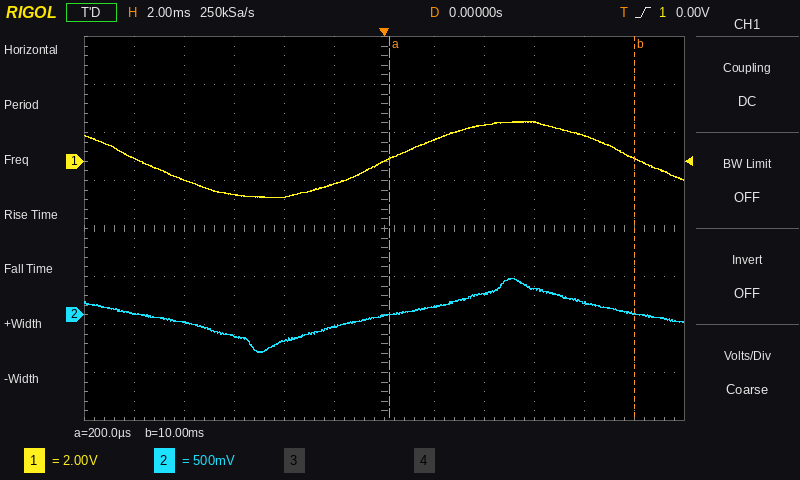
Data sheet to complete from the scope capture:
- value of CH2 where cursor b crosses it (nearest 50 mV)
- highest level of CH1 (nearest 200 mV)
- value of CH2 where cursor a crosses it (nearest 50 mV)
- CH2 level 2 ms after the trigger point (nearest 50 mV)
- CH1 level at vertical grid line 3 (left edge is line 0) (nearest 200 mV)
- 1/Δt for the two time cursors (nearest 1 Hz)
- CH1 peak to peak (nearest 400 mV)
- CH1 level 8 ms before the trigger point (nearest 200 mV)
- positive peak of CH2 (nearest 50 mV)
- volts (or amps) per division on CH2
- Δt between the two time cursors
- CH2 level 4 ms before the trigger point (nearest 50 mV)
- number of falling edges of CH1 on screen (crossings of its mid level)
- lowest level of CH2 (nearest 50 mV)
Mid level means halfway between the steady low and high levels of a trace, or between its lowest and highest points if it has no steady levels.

0 mV
1.6 V
0 mV
100 mV
-1.4 V
102 Hz
3.2 V
-800 mV
400 mV
500 mV
9.8 ms
-250 mV
2
-400 mV
